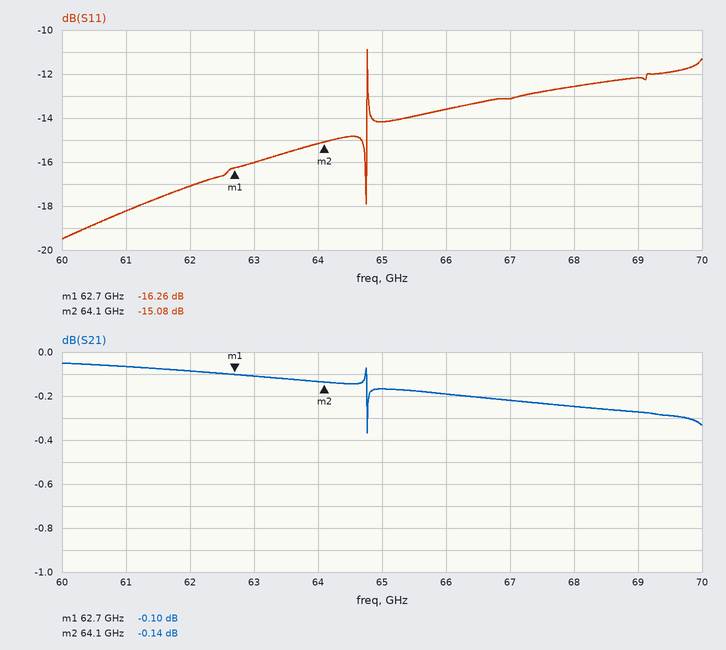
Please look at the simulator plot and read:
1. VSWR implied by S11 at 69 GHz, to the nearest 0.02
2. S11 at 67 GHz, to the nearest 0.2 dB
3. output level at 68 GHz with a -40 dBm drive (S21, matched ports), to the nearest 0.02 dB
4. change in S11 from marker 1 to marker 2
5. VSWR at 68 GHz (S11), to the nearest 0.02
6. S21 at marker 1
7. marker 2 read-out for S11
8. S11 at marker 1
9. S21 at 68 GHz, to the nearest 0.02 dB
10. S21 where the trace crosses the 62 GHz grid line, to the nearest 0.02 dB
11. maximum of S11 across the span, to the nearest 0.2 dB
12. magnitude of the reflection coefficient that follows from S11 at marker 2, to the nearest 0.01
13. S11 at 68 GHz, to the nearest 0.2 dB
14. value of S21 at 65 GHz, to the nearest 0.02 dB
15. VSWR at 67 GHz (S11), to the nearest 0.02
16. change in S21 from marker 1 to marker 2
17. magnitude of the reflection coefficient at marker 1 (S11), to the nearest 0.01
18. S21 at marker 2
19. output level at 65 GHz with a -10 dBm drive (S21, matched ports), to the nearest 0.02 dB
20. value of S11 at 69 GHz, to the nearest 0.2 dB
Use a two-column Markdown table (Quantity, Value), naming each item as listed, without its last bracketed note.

| Quantity | Value |
|---|---|
| VSWR implied by S11 at 69 GHz, to the nearest 0.02 | 1.66 |
| S11 at 67 GHz, to the nearest 0.2 dB | -13.2 dB |
| output level at 68 GHz with a -40 dBm drive (S21, matched ports), to the nearest 0.02 dB | -40.24 dBm |
| change in S11 from marker 1 to marker 2 | 1.18 dB |
| VSWR at 68 GHz (S11), to the nearest 0.02 | 1.62 |
| S21 at marker 1 | -0.10 dB |
| marker 2 read-out for S11 | -15.08 dB |
| S11 at marker 1 | -16.26 dB |
| S21 at 68 GHz, to the nearest 0.02 dB | -0.24 dB |
| S21 where the trace crosses the 62 GHz grid line, to the nearest 0.02 dB | -0.08 dB |
| maximum of S11 across the span, to the nearest 0.2 dB | -10.8 dB |
| magnitude of the reflection coefficient that follows from S11 at marker 2, to the nearest 0.01 | 0.18 |
| S11 at 68 GHz, to the nearest 0.2 dB | -12.6 dB |
| value of S21 at 65 GHz, to the nearest 0.02 dB | -0.16 dB |
| VSWR at 67 GHz (S11), to the nearest 0.02 | 1.56 |
| change in S21 from marker 1 to marker 2 | -0.04 dB |
| magnitude of the reflection coefficient at marker 1 (S11), to the nearest 0.01 | 0.15 |
| S21 at marker 2 | -0.14 dB |
| output level at 65 GHz with a -10 dBm drive (S21, matched ports), to the nearest 0.02 dB | -10.16 dBm |
| value of S11 at 69 GHz, to the nearest 0.2 dB | -12.2 dB |
